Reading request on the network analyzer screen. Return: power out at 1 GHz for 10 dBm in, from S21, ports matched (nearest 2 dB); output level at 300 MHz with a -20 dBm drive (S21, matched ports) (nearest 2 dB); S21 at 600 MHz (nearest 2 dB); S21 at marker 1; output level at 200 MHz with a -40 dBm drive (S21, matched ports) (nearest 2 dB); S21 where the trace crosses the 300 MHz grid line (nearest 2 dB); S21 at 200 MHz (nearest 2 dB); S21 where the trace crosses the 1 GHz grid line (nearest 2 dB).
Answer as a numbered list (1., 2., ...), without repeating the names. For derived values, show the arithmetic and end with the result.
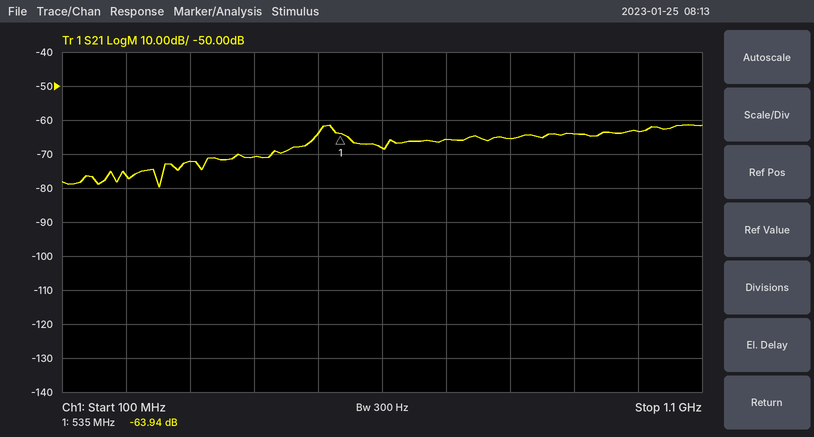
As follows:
1. 10 dBm + (-64 dB) = -54 dBm
2. -20 dBm + (-72 dB) = -92 dBm
3. -68 dB
4. -63.94 dB
5. -40 dBm + (-76 dB) = -116 dBm
6. -72 dB
7. -76 dB
8. -64 dB
